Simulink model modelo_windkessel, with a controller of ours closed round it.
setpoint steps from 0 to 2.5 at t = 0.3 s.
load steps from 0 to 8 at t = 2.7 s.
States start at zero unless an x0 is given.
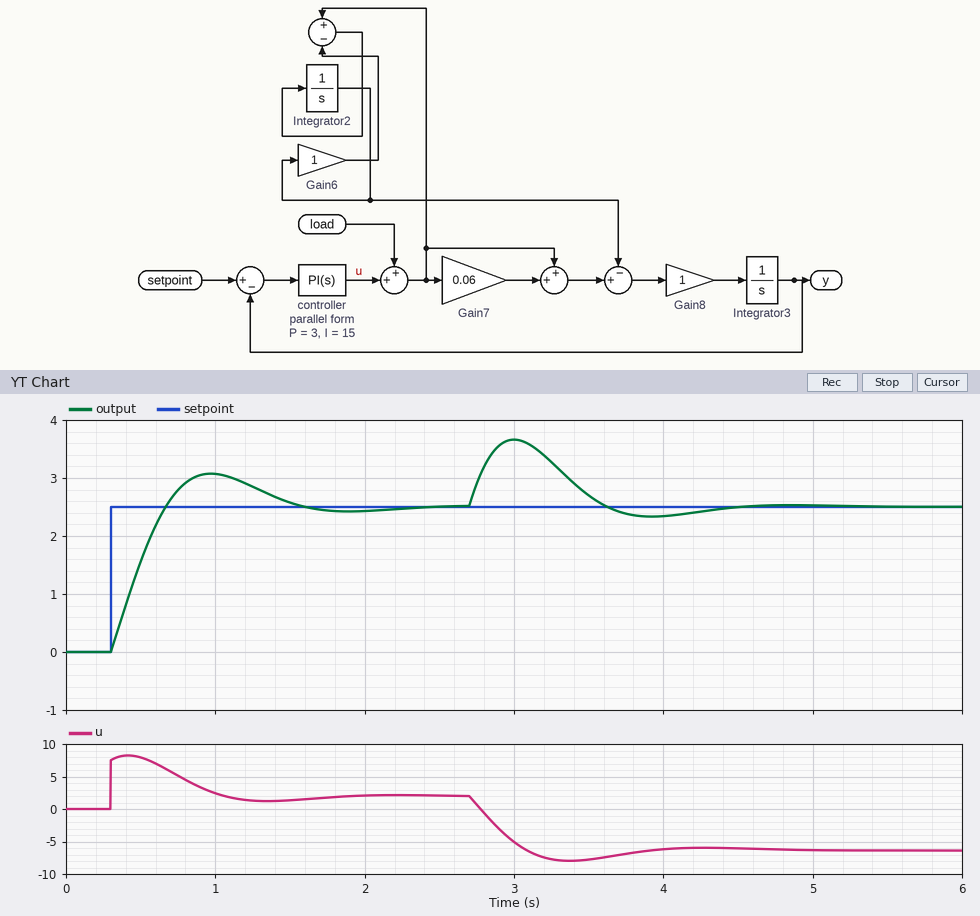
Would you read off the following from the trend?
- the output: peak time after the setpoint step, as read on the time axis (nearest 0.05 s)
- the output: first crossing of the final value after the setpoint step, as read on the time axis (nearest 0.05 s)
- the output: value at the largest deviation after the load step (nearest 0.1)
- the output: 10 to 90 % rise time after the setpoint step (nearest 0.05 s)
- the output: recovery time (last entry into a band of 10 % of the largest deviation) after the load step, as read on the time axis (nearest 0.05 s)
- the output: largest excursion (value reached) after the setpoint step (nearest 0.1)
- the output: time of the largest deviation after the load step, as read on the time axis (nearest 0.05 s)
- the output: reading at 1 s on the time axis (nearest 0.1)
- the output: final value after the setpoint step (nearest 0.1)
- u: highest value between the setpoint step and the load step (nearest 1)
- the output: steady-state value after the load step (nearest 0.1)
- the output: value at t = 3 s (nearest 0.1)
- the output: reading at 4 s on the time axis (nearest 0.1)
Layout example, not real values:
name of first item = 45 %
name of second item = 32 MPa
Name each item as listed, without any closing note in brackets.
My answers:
the output: peak time after the setpoint step, as read on the time axis = 0.95 s
the output: first crossing of the final value after the setpoint step, as read on the time axis = 0.65 s
the output: value at the largest deviation after the load step = 3.7
the output: 10 to 90 % rise time after the setpoint step = 0.30 s
the output: recovery time (last entry into a band of 10 % of the largest deviation) after the load step, as read on the time axis = 4.15 s
the output: largest excursion (value reached) after the setpoint step = 3.1
the output: time of the largest deviation after the load step, as read on the time axis = 3.00 s
the output: reading at 1 s on the time axis = 3.1
the output: final value after the setpoint step = 2.5
u: highest value between the setpoint step and the load step = 8
the output: steady-state value after the load step = 2.5
the output: value at t = 3 s = 3.7
the output: reading at 4 s on the time axis = 2.3
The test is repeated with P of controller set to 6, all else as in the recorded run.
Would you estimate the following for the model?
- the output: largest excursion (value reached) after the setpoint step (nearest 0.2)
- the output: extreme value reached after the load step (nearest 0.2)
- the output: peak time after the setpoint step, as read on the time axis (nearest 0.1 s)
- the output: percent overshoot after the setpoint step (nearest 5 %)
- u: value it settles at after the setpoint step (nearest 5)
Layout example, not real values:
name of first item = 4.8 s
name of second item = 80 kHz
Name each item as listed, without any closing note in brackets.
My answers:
the output: largest excursion (value reached) after the setpoint step = 2.8
the output: extreme value reached after the load step = 3.4
the output: peak time after the setpoint step, as read on the time axis = 0.9 s
the output: percent overshoot after the setpoint step = 10 %
u: value it settles at after the setpoint step = 0
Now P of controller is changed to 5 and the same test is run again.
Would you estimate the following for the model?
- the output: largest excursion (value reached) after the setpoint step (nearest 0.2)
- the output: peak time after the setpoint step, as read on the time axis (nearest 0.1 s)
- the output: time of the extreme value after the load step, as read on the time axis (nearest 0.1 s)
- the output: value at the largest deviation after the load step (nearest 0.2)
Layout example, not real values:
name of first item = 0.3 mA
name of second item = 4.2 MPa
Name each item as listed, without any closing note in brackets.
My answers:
the output: largest excursion (value reached) after the setpoint step = 2.8
the output: peak time after the setpoint step, as read on the time axis = 0.9 s
the output: time of the extreme value after the load step, as read on the time axis = 3.0 s
the output: value at the largest deviation after the load step = 3.4
